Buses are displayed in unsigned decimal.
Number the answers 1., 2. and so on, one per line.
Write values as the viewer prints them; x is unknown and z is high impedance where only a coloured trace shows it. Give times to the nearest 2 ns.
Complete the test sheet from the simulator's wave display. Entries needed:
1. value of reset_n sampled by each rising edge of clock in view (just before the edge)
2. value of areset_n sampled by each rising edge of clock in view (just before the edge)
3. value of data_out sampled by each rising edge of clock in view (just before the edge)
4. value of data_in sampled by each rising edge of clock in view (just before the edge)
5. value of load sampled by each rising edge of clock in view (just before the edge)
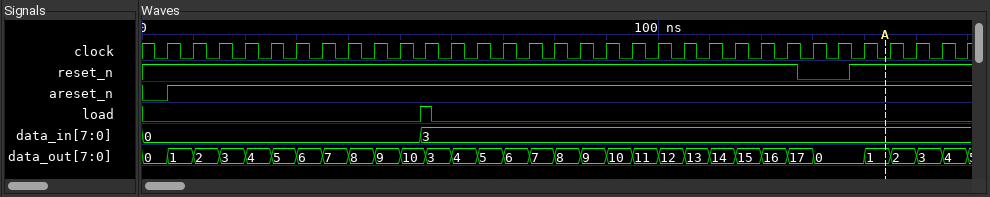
1. 1 1 1 1 1 1 1 1 1 1 1 1 1 1 1 1 1 1 1 1 1 1 1 1 1 0 0 1 1 1 1 1
2. 0 1 1 1 1 1 1 1 1 1 1 1 1 1 1 1 1 1 1 1 1 1 1 1 1 1 1 1 1 1 1 1
3. 0, 1, 2, 3, 4, 5, 6, 7, 8, 9, 10, 3, 4, 5, 6, 7, 8, 9, 10, 11, 12, 13, 14, 15, 16, 17, 0, 0, 1, 2, 3, 4
4. 0, 0, 0, 0, 0, 0, 0, 0, 0, 0, 3, 3, 3, 3, 3, 3, 3, 3, 3, 3, 3, 3, 3, 3, 3, 3, 3, 3, 3, 3, 3, 3
5. 0 0 0 0 0 0 0 0 0 0 1 0 0 0 0 0 0 0 0 0 0 0 0 0 0 0 0 0 0 0 0 0
